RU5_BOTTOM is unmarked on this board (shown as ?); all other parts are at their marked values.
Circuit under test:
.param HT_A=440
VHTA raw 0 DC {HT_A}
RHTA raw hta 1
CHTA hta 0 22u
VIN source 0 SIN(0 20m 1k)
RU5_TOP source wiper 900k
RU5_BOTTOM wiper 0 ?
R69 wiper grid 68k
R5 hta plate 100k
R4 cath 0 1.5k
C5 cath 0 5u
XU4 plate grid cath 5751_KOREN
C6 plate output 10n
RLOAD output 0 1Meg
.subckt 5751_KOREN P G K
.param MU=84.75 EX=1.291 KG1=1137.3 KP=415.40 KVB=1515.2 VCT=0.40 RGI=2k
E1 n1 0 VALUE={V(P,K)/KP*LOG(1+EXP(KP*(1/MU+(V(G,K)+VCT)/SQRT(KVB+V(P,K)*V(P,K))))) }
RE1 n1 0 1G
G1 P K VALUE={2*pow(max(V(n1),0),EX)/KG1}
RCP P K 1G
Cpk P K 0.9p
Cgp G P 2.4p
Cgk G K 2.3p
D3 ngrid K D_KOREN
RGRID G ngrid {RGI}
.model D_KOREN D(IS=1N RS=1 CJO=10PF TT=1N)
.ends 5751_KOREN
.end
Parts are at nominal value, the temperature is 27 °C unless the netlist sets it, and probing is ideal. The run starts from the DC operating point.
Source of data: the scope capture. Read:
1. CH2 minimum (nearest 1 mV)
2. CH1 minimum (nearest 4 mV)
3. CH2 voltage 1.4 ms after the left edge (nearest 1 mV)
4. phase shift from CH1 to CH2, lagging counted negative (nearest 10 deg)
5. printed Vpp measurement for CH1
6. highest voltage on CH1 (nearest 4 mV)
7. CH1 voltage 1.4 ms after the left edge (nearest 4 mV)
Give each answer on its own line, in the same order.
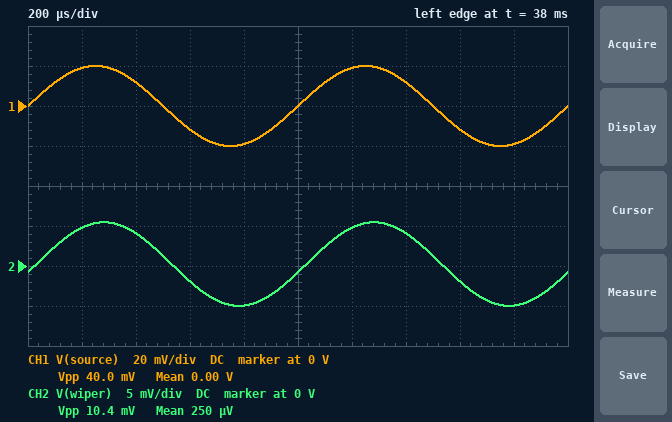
-5 mV
-20 mV
4 mV
-10 deg
40.0 mV
20 mV
12 mV
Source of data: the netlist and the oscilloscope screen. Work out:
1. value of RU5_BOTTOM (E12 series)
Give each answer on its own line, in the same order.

330 kΩ
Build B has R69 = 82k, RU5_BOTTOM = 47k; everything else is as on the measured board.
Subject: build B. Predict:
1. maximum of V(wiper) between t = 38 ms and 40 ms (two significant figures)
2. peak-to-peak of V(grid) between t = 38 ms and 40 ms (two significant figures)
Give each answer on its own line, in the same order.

1.0 mV
2.0 mV
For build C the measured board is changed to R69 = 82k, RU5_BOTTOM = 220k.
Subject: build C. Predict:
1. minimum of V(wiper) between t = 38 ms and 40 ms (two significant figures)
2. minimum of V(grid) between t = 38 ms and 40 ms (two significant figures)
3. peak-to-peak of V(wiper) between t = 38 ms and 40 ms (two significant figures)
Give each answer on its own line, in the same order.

-3.7 mV
-3.6 mV
7.7 mV
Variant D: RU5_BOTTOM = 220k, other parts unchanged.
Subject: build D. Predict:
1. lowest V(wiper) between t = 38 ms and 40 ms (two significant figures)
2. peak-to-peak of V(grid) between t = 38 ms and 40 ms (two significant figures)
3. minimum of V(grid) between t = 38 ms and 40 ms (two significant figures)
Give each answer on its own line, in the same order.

-3.7 mV
7.7 mV
-3.6 mV
